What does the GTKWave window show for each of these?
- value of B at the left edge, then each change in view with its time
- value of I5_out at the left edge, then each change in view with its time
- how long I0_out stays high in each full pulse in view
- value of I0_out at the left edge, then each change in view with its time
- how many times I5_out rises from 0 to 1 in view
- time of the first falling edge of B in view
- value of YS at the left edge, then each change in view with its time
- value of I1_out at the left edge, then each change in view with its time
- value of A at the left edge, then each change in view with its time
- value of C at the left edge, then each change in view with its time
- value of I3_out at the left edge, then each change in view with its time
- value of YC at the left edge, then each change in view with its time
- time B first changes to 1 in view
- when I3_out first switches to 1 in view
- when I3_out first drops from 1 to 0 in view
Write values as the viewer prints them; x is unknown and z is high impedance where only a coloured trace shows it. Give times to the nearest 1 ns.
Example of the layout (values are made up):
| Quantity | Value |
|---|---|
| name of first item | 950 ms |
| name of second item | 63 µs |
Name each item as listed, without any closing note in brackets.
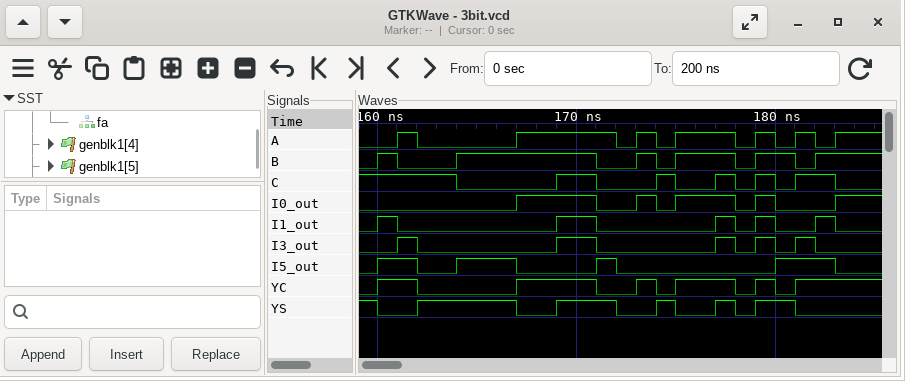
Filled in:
| Quantity | Value |
|---|---|
| value of B at the left edge, then each change in view with its time | 0, 1 at 160 ns, 0 at 161 ns, 1 at 164 ns, 0 at 171 ns, 1 at 173 ns, 0 at 174 ns, 1 at 175 ns, 0 at 178 ns, 1 at 179 ns, 0 at 181 ns, 1 at 182 ns |
| value of I5_out at the left edge, then each change in view with its time | 0, 1 at 160 ns, 0 at 162 ns, 1 at 164 ns, 0 at 167 ns, 1 at 171 ns, 0 at 172 ns, 1 at 180 ns, 0 at 183 ns |
| how long I0_out stays high in each full pulse in view | 4 ns, 1 ns, 3 ns, 1 ns |
| value of I0_out at the left edge, then each change in view with its time | 0, 1 at 167 ns, 0 at 171 ns, 1 at 173 ns, 0 at 174 ns, 1 at 175 ns, 0 at 178 ns, 1 at 179 ns, 0 at 180 ns, 1 at 183 ns |
| how many times I5_out rises from 0 to 1 in view | 4 |
| time of the first falling edge of B in view | 161 ns |
| value of YS at the left edge, then each change in view with its time | 1, 0 at 160 ns, 1 at 162 ns, 0 at 167 ns, 1 at 169 ns, 0 at 172 ns, 1 at 174 ns, 0 at 175 ns, 1 at 177 ns, 0 at 178 ns, 1 at 179 ns, 0 at 181 ns |
| value of I1_out at the left edge, then each change in view with its time | 0, 1 at 160 ns, 0 at 161 ns, 1 at 169 ns, 0 at 171 ns, 1 at 177 ns, 0 at 178 ns, 1 at 179 ns, 0 at 180 ns, 1 at 182 ns, 0 at 183 ns |
| value of A at the left edge, then each change in view with its time | 0, 1 at 161 ns, 0 at 162 ns, 1 at 167 ns, 0 at 172 ns, 1 at 173 ns, 0 at 174 ns, 1 at 175 ns, 0 at 178 ns, 1 at 179 ns, 0 at 180 ns, 1 at 181 ns, 0 at 182 ns, 1 at 183 ns |
| value of C at the left edge, then each change in view with its time | 1, 0 at 164 ns, 1 at 169 ns, 0 at 171 ns, 1 at 174 ns, 0 at 175 ns, 1 at 177 ns, 0 at 178 ns, 1 at 179 ns, 0 at 180 ns, 1 at 181 ns, 0 at 183 ns |
| value of I3_out at the left edge, then each change in view with its time | 0, 1 at 161 ns, 0 at 162 ns, 1 at 169 ns, 0 at 171 ns, 1 at 177 ns, 0 at 178 ns, 1 at 179 ns, 0 at 180 ns, 1 at 181 ns, 0 at 182 ns |
| value of YC at the left edge, then each change in view with its time | 0, 1 at 160 ns, 0 at 162 ns, 1 at 167 ns, 0 at 171 ns, 1 at 173 ns, 0 at 174 ns, 1 at 175 ns, 0 at 178 ns, 1 at 179 ns, 0 at 180 ns, 1 at 181 ns |
| time B first changes to 1 in view | 160 ns |
| when I3_out first switches to 1 in view | 161 ns |
| when I3_out first drops from 1 to 0 in view | 162 ns |
